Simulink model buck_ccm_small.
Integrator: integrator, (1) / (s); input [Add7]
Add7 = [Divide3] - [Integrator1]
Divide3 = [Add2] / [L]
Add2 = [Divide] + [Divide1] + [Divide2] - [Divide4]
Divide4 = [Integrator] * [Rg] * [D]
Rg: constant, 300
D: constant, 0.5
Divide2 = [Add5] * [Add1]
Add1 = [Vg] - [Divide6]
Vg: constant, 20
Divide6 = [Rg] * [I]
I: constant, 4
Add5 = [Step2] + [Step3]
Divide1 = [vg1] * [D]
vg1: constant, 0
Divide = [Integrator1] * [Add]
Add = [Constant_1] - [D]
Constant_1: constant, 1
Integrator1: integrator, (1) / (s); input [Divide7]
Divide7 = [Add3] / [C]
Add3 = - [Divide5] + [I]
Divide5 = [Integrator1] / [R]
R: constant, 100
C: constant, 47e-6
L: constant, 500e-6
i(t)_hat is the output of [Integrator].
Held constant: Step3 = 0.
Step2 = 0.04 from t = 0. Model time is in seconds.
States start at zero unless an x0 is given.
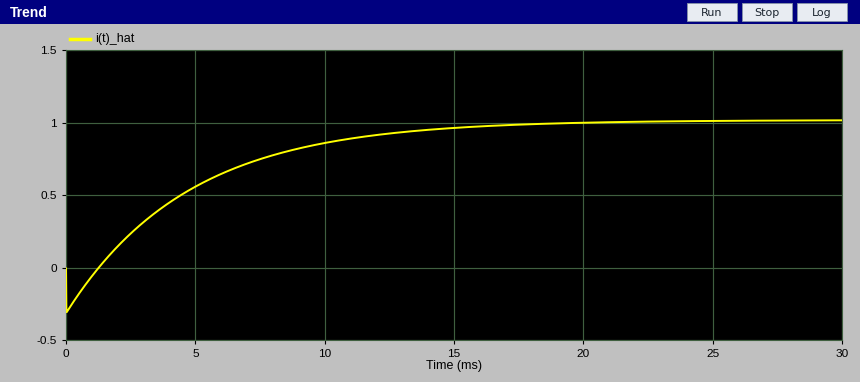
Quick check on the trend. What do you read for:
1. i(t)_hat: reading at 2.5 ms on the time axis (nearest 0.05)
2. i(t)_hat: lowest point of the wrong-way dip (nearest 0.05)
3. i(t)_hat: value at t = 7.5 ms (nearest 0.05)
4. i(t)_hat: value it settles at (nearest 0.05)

0.25
-0.30
0.75
1.00
